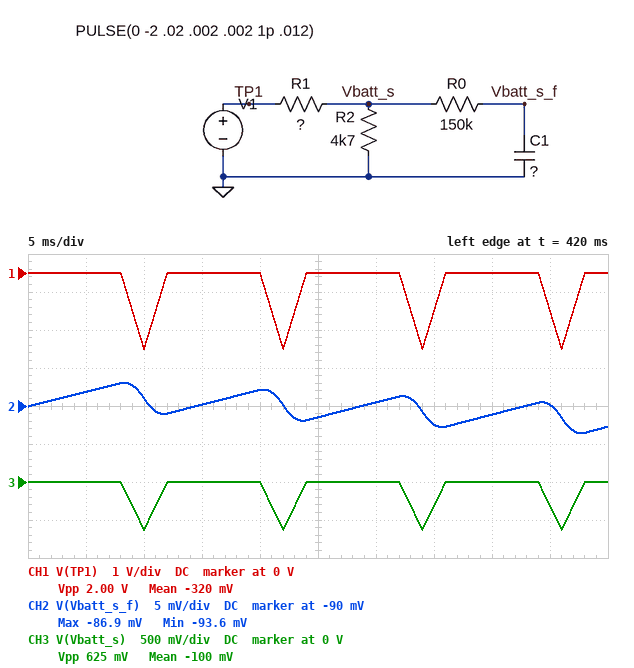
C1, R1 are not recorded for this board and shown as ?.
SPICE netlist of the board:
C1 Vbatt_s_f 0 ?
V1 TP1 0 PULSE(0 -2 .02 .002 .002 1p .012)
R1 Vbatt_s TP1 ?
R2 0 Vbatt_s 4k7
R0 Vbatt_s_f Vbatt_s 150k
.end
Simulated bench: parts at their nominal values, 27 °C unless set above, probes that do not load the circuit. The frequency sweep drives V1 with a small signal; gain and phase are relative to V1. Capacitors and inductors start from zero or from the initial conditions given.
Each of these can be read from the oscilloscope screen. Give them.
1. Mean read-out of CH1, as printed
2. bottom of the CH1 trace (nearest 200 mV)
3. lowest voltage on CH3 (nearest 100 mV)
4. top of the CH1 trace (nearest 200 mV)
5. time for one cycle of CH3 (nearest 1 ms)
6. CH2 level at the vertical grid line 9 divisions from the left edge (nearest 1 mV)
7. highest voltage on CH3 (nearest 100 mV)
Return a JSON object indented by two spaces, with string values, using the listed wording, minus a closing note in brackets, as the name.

{
  "Mean read-out of CH1, as printed": "-320 mV",
  "bottom of the CH1 trace": "-2.0 V",
  "lowest voltage on CH3": "-600 mV",
  "top of the CH1 trace": "0 V",
  "time for one cycle of CH3": "12 ms",
  "CH2 level at the vertical grid line 9 divisions from the left edge": "-90 mV",
  "highest voltage on CH3": "0 V"
}
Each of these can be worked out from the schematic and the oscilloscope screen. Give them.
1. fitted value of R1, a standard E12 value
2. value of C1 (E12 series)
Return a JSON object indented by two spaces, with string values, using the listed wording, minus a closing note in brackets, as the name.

{
  "fitted value of R1, a standard E12 value": "10 kΩ",
  "value of C1": "1.5 µF"
}
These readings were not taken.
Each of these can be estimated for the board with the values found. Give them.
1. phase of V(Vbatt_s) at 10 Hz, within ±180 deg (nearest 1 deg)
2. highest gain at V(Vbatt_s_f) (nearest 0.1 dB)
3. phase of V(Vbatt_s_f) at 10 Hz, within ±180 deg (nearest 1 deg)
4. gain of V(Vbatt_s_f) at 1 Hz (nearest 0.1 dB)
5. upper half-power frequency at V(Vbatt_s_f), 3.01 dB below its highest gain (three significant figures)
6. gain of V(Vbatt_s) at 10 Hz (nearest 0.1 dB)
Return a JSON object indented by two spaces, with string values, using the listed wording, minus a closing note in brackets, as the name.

{
  "phase of V(Vbatt_s) at 10 Hz, within ±180 deg": "0 deg",
  "highest gain at V(Vbatt_s_f)": "-9.9 dB",
  "phase of V(Vbatt_s_f) at 10 Hz, within ±180 deg": "-86 deg",
  "gain of V(Vbatt_s_f) at 1 Hz": "-14.8 dB",
  "upper half-power frequency at V(Vbatt_s_f), 3.01 dB below its highest gain": "693 mHz",
  "gain of V(Vbatt_s) at 10 Hz": "-10.1 dB"
}
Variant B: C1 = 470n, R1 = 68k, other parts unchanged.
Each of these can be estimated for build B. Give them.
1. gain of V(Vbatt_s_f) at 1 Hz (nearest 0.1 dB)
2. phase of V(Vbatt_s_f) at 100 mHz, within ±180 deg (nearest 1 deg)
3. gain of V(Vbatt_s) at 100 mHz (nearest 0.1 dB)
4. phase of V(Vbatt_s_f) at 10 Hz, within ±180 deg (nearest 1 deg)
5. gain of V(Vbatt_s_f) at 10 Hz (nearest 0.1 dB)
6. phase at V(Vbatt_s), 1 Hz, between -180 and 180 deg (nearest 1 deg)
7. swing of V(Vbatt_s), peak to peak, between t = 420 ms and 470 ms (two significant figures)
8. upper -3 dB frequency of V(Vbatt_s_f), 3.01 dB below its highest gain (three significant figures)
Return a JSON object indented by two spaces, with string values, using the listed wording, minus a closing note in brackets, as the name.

{
  "gain of V(Vbatt_s_f) at 1 Hz": "-24.6 dB",
  "phase of V(Vbatt_s_f) at 100 mHz, within ±180 deg": "-3 deg",
  "gain of V(Vbatt_s) at 100 mHz": "-23.8 dB",
  "phase of V(Vbatt_s_f) at 10 Hz, within ±180 deg": "-78 deg",
  "gain of V(Vbatt_s_f) at 10 Hz": "-37.2 dB",
  "phase at V(Vbatt_s), 1 Hz, between -180 and 180 deg": "-1 deg",
  "swing of V(Vbatt_s), peak to peak, between t = 420 ms and 470 ms": "130 mV",
  "upper -3 dB frequency of V(Vbatt_s_f), 3.01 dB below its highest gain": "2.19 Hz"
}
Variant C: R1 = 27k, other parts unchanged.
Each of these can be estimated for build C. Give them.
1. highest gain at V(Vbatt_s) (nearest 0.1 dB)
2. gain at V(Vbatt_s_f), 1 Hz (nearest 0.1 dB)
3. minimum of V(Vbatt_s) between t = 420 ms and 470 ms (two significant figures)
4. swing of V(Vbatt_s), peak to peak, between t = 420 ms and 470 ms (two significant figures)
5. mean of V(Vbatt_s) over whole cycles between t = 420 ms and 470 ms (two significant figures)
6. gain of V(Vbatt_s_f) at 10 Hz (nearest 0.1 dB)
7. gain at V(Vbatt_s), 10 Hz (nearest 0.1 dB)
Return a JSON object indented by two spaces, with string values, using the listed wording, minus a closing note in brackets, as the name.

{
  "highest gain at V(Vbatt_s)": "-16.6 dB",
  "gain at V(Vbatt_s_f), 1 Hz": "-21.5 dB",
  "minimum of V(Vbatt_s) between t = 420 ms and 470 ms": "-290 mV",
  "swing of V(Vbatt_s), peak to peak, between t = 420 ms and 470 ms": "290 mV",
  "mean of V(Vbatt_s) over whole cycles between t = 420 ms and 470 ms": "-49 mV",
  "gain of V(Vbatt_s_f) at 10 Hz": "-39.8 dB",
  "gain at V(Vbatt_s), 10 Hz": "-16.8 dB"
}
